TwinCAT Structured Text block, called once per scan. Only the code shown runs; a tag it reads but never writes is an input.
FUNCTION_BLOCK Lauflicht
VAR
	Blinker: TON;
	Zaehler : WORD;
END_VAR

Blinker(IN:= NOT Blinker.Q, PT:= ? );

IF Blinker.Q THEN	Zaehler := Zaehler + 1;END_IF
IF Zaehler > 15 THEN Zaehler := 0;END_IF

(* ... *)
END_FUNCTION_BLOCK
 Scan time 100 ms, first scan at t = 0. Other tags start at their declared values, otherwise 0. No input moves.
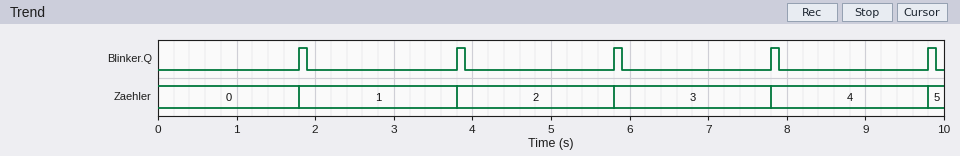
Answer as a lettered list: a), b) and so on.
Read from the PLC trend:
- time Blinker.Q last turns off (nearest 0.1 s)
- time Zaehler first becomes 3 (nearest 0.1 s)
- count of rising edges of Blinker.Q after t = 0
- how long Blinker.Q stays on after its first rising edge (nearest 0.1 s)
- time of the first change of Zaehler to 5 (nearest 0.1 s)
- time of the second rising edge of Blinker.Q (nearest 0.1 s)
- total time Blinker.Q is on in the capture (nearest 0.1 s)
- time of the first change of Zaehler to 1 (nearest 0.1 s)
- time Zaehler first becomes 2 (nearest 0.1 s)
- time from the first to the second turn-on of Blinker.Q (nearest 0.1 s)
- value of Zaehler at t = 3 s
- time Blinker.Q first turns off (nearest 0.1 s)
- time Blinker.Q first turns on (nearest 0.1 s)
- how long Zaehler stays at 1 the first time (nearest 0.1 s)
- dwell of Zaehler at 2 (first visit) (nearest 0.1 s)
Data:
a) 9.9 s
b) 5.8 s
c) 5
d) 0.1 s
e) 9.8 s
f) 3.8 s
g) 0.5 s
h) 1.8 s
i) 3.8 s
j) 2.0 s
k) 1
l) 1.9 s
m) 1.8 s
n) 2.0 s
o) 2.0 s
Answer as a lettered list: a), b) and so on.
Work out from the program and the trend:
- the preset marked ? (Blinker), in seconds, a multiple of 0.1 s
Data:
a) 1.8 s
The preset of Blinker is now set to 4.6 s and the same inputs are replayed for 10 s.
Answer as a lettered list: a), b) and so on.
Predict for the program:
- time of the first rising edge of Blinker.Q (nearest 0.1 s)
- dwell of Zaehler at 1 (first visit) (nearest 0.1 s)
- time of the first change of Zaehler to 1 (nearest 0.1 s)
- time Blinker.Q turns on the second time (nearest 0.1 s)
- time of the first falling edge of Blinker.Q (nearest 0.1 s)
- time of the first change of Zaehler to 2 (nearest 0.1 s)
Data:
a) 4.6 s
b) 4.8 s
c) 4.6 s
d) 9.4 s
e) 4.7 s
f) 9.4 s
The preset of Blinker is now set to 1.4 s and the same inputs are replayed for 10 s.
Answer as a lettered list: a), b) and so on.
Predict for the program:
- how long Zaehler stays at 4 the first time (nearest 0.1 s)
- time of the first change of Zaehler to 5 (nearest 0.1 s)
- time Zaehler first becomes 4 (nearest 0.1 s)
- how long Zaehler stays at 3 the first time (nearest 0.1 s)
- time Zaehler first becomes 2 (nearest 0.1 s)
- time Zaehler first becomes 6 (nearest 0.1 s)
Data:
a) 1.6 s
b) 7.8 s
c) 6.2 s
d) 1.6 s
e) 3.0 s
f) 9.4 s
